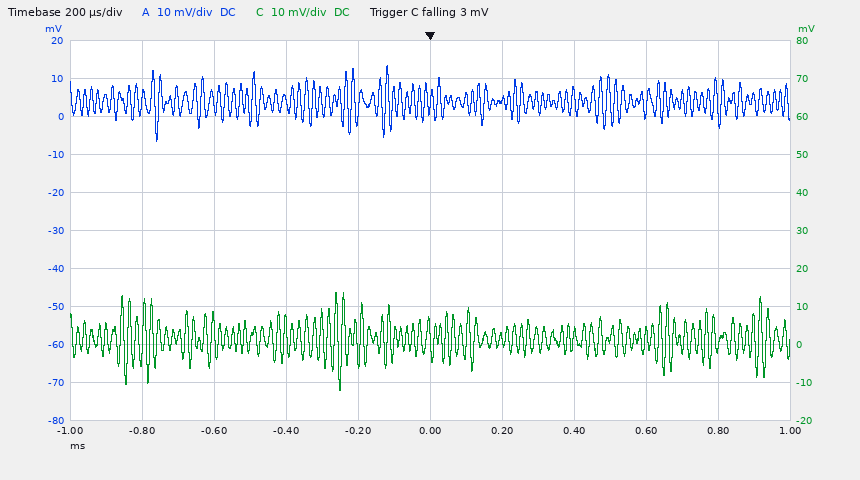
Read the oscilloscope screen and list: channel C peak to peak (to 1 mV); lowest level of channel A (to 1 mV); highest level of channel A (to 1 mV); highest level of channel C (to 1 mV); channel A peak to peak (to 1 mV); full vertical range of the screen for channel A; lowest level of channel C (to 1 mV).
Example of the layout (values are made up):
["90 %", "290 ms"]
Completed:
["26 mV", "-7 mV", "13 mV", "14 mV", "20 mV", "100 mV", "-12 mV"]
